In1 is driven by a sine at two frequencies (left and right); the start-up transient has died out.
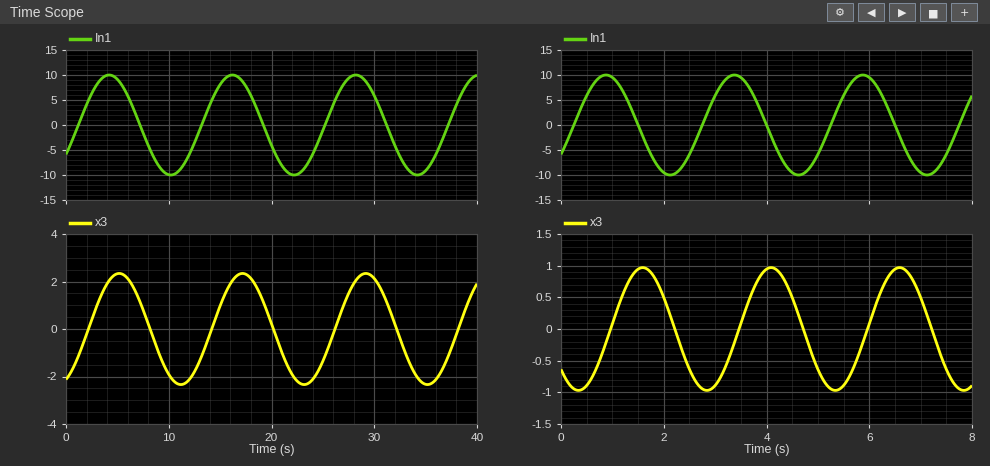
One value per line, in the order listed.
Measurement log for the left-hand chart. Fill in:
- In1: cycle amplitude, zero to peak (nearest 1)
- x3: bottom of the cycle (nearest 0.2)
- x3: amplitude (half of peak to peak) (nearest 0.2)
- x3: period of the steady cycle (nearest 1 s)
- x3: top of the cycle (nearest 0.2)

10
-2.4
2.4
12 s
2.4
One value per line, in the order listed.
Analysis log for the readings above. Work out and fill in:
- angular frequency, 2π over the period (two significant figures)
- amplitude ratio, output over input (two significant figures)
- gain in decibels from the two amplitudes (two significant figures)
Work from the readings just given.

0.52 rad/s
0.24
-12 dB
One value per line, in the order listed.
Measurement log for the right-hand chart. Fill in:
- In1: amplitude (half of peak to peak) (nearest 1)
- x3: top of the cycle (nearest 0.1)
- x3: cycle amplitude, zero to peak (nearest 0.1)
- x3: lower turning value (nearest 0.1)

10
1.0
1.0
-1.0
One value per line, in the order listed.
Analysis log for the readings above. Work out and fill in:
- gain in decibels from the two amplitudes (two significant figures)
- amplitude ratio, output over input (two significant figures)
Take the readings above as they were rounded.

-20 dB
0.10
